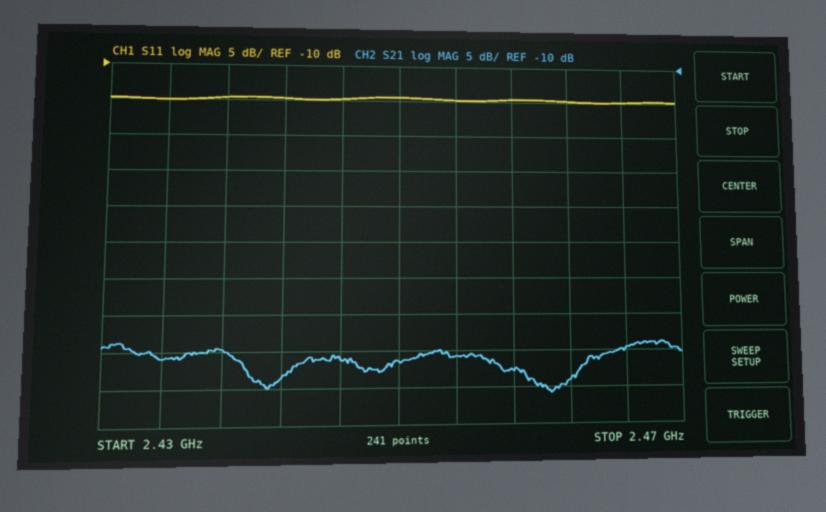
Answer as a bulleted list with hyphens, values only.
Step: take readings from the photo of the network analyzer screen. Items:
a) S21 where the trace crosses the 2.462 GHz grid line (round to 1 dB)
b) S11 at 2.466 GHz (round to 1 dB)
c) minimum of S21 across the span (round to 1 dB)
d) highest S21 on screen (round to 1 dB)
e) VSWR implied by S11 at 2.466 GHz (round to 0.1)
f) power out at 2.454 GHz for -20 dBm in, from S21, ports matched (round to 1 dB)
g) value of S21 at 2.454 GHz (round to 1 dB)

- -54 dB
- -15 dB
- -56 dB
- -49 dB
- 1.4
- -71 dBm
- -51 dB
